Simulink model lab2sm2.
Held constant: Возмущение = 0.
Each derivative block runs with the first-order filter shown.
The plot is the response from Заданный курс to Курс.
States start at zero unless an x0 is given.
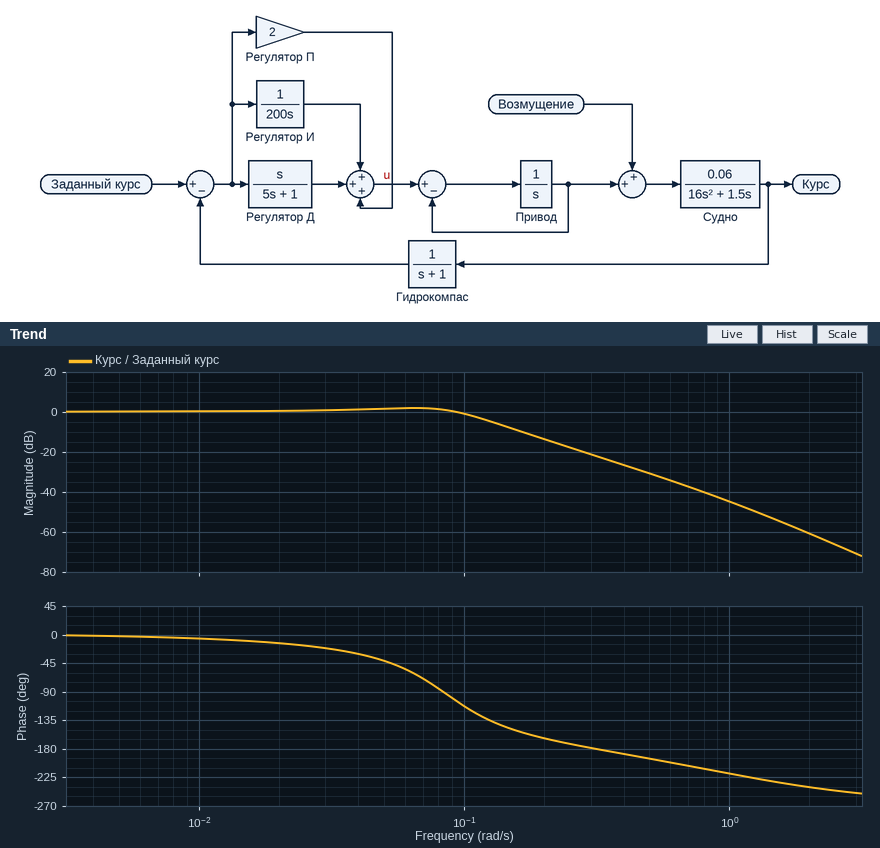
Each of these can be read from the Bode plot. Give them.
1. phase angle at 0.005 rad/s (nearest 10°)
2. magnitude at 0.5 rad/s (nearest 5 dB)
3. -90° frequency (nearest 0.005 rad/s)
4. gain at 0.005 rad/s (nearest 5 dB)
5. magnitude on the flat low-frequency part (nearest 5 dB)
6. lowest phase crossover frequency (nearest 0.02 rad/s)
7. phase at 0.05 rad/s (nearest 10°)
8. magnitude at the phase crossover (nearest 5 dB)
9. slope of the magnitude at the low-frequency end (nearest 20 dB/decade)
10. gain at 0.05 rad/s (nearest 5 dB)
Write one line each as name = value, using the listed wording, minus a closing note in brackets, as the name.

phase angle at 0.005 rad/s = 0°
magnitude at 0.5 rad/s = -30 dB
-90° frequency = 0.085 rad/s
gain at 0.005 rad/s = 0 dB
magnitude on the flat low-frequency part = 0 dB
lowest phase crossover frequency = 0.32 rad/s
phase at 0.05 rad/s = -40°
magnitude at the phase crossover = -20 dB
slope of the magnitude at the low-frequency end = 0 dB/decade
gain at 0.05 rad/s = 0 dB
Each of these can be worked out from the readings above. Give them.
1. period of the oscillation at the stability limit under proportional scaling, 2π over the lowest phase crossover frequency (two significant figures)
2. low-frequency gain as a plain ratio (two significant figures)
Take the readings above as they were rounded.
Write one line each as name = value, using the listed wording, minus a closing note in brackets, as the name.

period of the oscillation at the stability limit under proportional scaling, 2π over the lowest phase crossover frequency = 20 s
low-frequency gain as a plain ratio = 1.0
